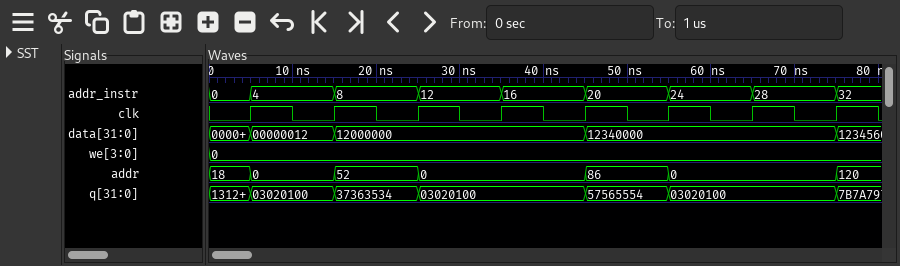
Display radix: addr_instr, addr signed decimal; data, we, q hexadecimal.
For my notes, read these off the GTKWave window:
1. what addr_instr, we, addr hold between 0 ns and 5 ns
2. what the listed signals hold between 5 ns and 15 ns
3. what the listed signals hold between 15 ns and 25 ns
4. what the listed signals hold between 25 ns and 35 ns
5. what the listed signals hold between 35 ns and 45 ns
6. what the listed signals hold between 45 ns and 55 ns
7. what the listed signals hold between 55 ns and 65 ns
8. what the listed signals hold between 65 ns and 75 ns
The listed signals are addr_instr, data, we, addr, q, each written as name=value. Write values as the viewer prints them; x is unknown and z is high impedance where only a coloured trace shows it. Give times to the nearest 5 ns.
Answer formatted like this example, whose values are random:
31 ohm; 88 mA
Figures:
addr_instr=0, we=0, addr=18; addr_instr=4, data=00000012, we=0, addr=0, q=03020100; addr_instr=8, data=12000000, we=0, addr=52, q=37363534; addr_instr=12, data=12000000, we=0, addr=0, q=03020100; addr_instr=16, data=12000000, we=0, addr=0, q=03020100; addr_instr=20, data=12340000, we=0, addr=86, q=57565554; addr_instr=24, data=12340000, we=0, addr=0, q=03020100; addr_instr=28, data=12340000, we=0, addr=0, q=03020100
